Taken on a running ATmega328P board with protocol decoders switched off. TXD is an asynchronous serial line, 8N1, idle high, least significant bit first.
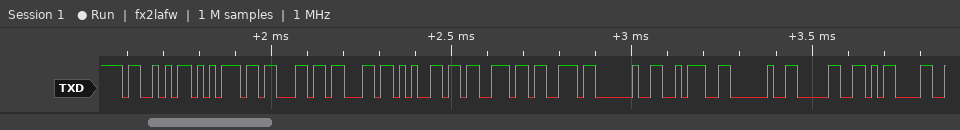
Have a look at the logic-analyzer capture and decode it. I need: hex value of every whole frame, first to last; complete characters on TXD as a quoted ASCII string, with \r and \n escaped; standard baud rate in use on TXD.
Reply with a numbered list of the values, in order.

1. 0x53 0x75 0x63 0x63 0x65 0x73 0x73 0x20 0x3A 0x20 0x30 0x0D
2. "Success : 0\r"
3. 57600 baud
